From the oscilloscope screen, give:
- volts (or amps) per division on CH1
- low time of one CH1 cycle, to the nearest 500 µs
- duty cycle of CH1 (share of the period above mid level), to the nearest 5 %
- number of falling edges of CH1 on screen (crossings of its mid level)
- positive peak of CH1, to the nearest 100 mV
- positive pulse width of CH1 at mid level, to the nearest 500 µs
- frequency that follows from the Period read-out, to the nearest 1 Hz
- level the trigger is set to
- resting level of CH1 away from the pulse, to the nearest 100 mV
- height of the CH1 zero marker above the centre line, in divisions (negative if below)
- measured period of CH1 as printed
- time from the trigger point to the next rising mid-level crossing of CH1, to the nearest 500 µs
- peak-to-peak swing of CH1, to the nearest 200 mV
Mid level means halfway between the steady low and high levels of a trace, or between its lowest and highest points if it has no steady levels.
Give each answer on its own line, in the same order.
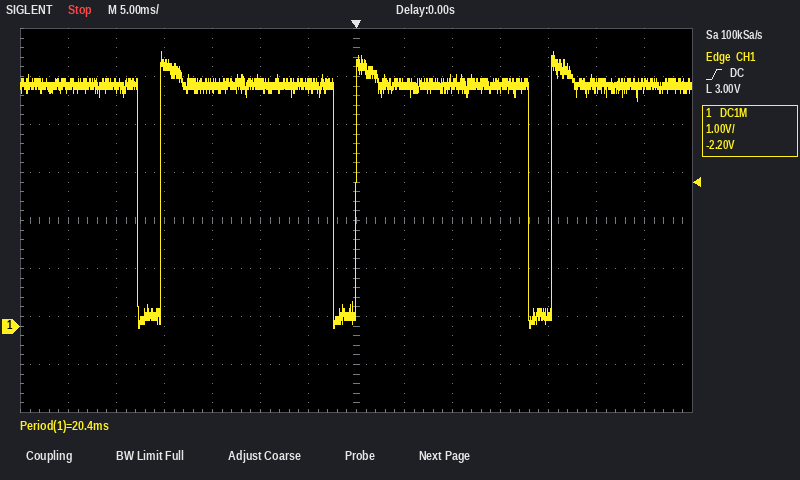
1 V
2.5 ms
90 %
3
5.7 V
18.0 ms
49 Hz
3.00 V
5.0 V
-2.2 div
20.4 ms
20.5 ms
5.8 V
